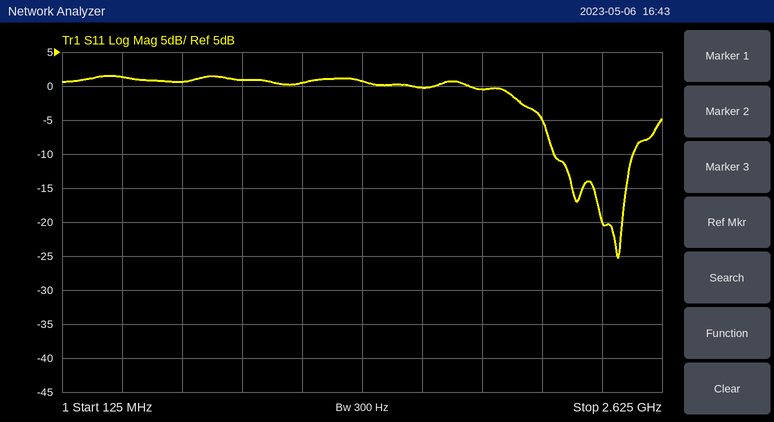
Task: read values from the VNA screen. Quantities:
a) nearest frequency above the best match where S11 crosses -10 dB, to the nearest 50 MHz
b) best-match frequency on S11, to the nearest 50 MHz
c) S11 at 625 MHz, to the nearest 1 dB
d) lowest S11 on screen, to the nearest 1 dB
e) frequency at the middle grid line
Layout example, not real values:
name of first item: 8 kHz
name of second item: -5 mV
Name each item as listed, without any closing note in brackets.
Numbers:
nearest frequency above the best match where S11 crosses -10 dB, to the nearest 50 MHz: 2.50 GHz
best-match frequency on S11, to the nearest 50 MHz: 2.45 GHz
S11 at 625 MHz, to the nearest 1 dB: 1 dB
lowest S11 on screen, to the nearest 1 dB: -25 dB
frequency at the middle grid line: 1.375 GHz
